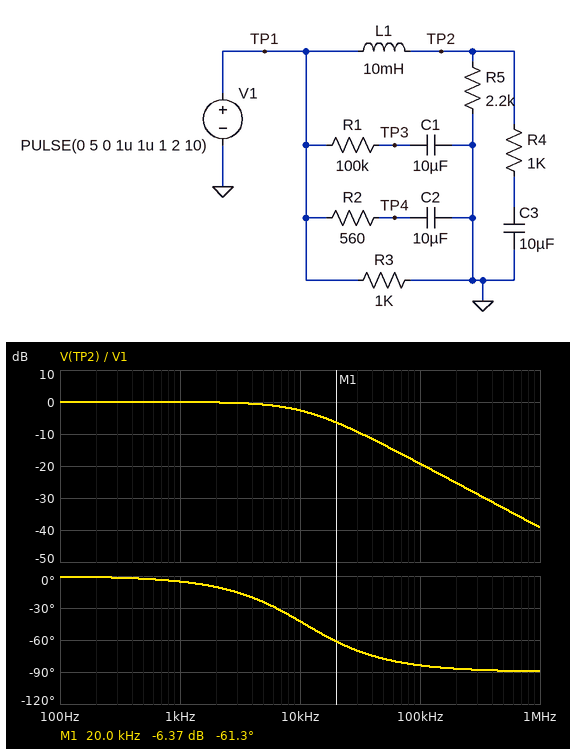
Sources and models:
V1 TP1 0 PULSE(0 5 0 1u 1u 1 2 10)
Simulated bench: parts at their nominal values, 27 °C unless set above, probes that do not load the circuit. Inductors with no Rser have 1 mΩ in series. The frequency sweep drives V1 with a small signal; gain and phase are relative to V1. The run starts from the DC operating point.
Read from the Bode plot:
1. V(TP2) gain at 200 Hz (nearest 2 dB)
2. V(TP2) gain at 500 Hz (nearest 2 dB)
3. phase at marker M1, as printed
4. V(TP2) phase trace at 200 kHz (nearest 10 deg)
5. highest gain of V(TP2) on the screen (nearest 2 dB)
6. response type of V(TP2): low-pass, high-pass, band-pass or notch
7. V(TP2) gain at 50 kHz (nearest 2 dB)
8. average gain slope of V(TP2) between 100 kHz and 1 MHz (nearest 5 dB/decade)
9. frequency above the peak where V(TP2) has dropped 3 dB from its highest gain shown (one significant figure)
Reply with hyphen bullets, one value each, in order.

- 0 dB
- 0 dB
- -61.3 deg
- -90 deg
- 0 dB
- low-pass
- -14 dB
- -20 dB/decade
- 10 kHz
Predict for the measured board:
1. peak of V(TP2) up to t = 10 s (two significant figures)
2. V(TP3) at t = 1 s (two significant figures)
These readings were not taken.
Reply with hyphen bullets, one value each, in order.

- 5.0 V
- 3.2 V
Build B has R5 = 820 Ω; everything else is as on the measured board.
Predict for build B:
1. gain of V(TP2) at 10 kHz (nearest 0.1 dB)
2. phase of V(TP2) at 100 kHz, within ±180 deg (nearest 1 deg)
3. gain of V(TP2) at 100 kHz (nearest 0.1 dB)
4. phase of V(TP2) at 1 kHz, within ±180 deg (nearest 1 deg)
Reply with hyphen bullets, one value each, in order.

- -4.7 dB
- -86 deg
- -22.9 dB
- -8 deg
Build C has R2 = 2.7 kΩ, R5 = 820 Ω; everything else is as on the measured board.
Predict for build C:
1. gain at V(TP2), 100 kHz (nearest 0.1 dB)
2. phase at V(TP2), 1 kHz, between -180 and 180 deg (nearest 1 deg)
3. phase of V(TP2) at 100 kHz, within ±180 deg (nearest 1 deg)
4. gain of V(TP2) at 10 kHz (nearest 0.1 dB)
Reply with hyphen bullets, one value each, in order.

- -22.9 dB
- -8 deg
- -86 deg
- -4.7 dB
